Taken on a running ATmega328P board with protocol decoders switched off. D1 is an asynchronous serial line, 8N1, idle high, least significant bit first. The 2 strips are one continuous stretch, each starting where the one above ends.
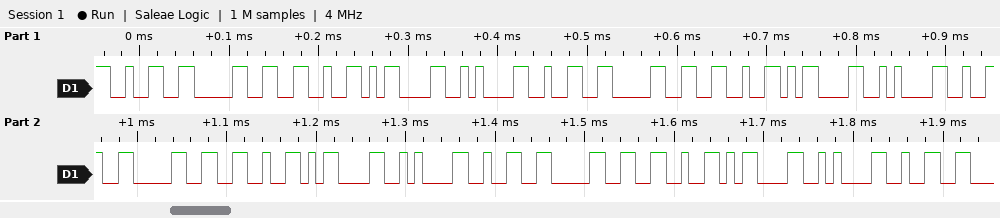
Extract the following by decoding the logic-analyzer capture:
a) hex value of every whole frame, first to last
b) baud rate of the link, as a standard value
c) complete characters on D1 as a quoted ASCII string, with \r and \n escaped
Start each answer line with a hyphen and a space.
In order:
- 32 30 26 0D 0A 32 30 26 0D 0A 32 30 26 0D 0A 32 30 26 0D 0A 32
- 115200 baud
- "20&\r\n20&\r\n20&\r\n20&\r\n2"
